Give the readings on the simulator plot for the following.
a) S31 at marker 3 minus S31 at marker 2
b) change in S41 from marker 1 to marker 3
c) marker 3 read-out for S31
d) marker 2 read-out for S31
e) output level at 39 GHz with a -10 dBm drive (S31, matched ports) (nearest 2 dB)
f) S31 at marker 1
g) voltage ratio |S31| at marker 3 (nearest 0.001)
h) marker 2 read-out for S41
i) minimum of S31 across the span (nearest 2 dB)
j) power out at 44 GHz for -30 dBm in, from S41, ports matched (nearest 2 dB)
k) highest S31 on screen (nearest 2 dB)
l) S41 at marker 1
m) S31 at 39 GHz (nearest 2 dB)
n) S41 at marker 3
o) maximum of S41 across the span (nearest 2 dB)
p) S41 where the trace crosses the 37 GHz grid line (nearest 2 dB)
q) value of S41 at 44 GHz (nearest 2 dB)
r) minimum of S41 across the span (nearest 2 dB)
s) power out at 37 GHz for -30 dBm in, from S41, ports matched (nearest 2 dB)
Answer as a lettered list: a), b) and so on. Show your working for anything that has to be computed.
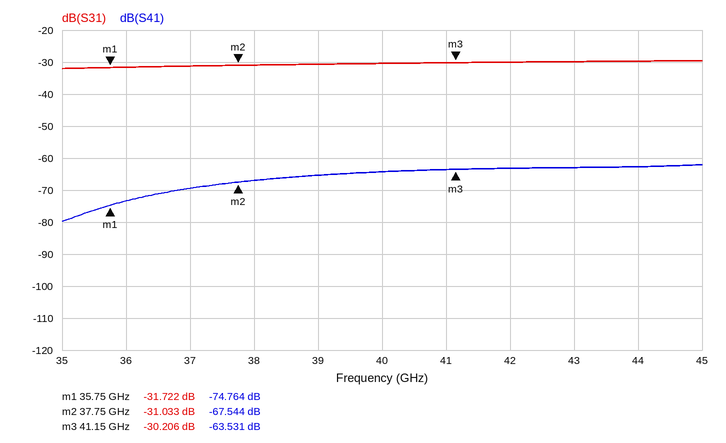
a) -30.206 − (-31.033) = 0.827 dB
b) -63.531 − (-74.764) = 11.233 dB
c) -30.206 dB
d) -31.033 dB
e) -10 dBm + (-30 dB) = -40 dBm
f) -31.722 dB
g) 10^(-30.206/20) ≈ 0.031
h) -67.544 dB
i) -32 dB
j) -30 dBm + (-62 dB) = -92 dBm
k) -30 dB
l) -74.764 dB
m) -30 dB
n) -63.531 dB
o) -62 dB
p) -70 dB
q) -62 dB
r) -80 dB
s) -30 dBm + (-70 dB) = -100 dBm
